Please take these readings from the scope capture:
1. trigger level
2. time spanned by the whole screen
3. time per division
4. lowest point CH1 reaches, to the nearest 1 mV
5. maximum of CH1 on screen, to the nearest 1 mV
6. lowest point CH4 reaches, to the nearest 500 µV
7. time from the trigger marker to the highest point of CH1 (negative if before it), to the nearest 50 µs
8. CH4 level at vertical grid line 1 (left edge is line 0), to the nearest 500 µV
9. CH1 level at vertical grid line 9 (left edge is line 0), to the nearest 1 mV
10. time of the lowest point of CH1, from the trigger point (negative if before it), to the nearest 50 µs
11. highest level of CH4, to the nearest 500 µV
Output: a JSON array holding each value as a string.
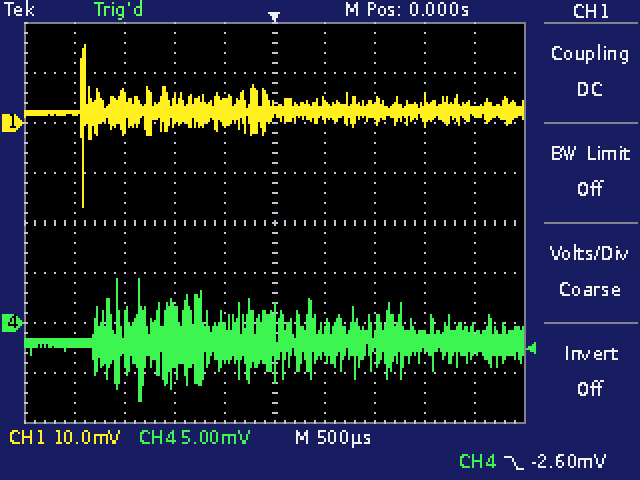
["-2.60 mV", "5 ms", "500 µs", "-17 mV", "16 mV", "-8.0 mV", "-1.90 ms", "-2.0 mV", "2 mV", "-1.90 ms", "4.5 mV"]
